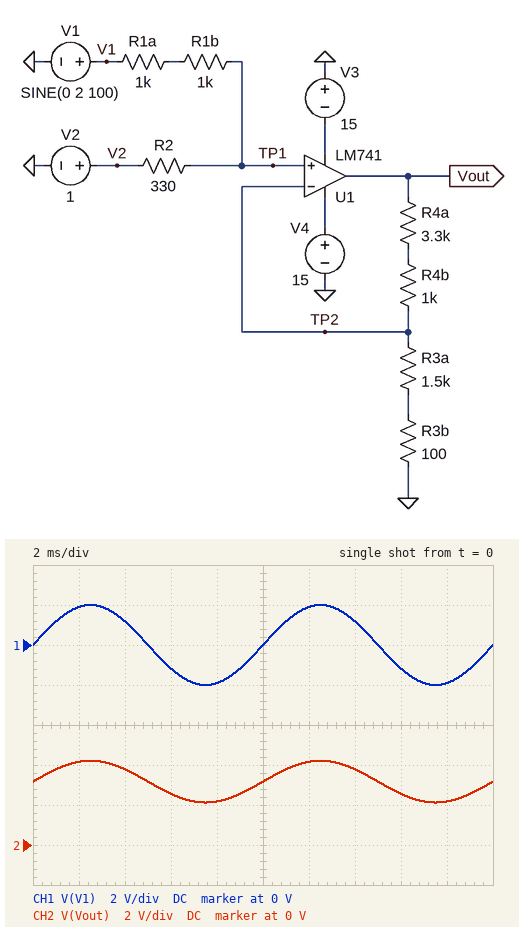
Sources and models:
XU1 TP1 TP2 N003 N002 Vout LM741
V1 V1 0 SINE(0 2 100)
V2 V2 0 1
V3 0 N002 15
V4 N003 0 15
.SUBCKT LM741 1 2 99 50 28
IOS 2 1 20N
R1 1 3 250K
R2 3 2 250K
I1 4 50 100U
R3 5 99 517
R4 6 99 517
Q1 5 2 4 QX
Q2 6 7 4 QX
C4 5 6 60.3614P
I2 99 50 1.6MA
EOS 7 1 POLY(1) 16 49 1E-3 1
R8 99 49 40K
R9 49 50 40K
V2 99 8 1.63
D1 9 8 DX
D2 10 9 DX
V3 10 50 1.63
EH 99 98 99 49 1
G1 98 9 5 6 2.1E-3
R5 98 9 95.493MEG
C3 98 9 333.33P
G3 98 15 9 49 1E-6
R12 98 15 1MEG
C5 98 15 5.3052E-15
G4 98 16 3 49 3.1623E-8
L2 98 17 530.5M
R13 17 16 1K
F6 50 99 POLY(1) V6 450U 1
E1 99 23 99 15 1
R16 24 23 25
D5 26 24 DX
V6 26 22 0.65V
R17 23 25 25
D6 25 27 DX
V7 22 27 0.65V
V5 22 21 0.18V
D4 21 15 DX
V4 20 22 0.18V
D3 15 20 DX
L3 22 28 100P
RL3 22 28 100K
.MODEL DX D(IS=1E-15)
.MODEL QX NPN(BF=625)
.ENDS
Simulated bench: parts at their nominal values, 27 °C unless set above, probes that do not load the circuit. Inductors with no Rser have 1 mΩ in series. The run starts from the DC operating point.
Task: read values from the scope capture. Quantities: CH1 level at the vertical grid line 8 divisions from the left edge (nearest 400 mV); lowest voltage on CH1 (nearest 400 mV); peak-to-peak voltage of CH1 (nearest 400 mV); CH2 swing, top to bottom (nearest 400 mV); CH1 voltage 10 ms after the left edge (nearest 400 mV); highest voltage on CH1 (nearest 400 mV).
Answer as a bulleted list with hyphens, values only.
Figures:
- -1.2 V
- -2.0 V
- 4.0 V
- 2.0 V
- 0 V
- 2.0 V
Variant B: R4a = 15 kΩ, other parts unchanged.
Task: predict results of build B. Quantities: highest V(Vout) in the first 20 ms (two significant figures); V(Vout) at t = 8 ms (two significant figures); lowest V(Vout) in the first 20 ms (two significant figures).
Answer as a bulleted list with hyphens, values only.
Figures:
- 13 V
- 6.5 V
- 6.3 V
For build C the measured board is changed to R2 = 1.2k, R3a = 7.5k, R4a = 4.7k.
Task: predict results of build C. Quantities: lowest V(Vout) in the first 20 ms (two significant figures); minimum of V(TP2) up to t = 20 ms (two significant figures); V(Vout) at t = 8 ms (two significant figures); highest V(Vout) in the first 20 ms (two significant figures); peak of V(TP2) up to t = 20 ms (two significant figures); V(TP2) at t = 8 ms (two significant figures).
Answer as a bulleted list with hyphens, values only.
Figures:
- -220 mV
- -120 mV
- -150 mV
- 2.4 V
- 1.4 V
- -87 mV
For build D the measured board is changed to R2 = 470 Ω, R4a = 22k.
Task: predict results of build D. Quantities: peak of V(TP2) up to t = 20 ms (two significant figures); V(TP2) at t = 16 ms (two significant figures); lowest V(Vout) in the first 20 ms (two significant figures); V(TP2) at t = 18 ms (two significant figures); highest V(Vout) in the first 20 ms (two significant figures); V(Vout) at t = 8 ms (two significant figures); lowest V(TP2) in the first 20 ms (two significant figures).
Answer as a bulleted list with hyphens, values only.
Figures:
- 910 mV
- 590 mV
- 6.6 V
- 450 mV
- 14 V
- 6.9 V
- 430 mV
